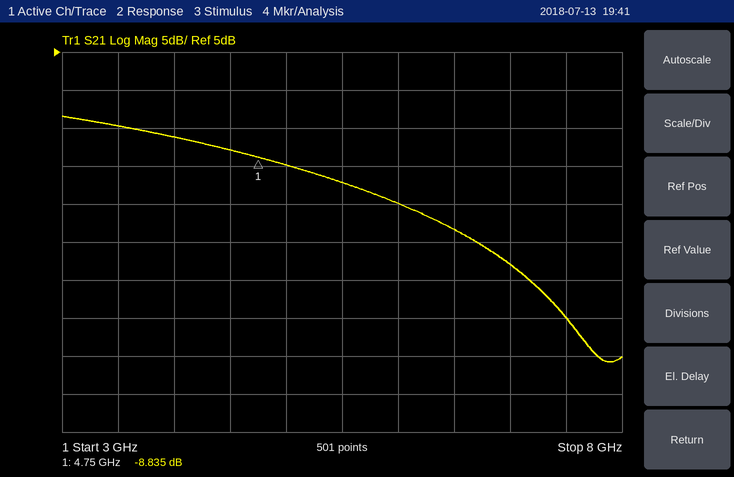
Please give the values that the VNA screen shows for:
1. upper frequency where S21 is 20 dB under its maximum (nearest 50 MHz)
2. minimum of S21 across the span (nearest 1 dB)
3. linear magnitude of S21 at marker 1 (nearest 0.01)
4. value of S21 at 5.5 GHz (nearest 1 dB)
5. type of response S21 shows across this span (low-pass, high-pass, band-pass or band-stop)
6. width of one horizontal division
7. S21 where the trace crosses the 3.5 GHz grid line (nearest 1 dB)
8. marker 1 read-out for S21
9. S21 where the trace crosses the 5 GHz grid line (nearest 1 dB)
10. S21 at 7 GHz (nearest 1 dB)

7.05 GHz
-36 dB
0.36
-12 dB
low-pass
500 MHz
-5 dB
-8.835 dB
-10 dB
-23 dB
